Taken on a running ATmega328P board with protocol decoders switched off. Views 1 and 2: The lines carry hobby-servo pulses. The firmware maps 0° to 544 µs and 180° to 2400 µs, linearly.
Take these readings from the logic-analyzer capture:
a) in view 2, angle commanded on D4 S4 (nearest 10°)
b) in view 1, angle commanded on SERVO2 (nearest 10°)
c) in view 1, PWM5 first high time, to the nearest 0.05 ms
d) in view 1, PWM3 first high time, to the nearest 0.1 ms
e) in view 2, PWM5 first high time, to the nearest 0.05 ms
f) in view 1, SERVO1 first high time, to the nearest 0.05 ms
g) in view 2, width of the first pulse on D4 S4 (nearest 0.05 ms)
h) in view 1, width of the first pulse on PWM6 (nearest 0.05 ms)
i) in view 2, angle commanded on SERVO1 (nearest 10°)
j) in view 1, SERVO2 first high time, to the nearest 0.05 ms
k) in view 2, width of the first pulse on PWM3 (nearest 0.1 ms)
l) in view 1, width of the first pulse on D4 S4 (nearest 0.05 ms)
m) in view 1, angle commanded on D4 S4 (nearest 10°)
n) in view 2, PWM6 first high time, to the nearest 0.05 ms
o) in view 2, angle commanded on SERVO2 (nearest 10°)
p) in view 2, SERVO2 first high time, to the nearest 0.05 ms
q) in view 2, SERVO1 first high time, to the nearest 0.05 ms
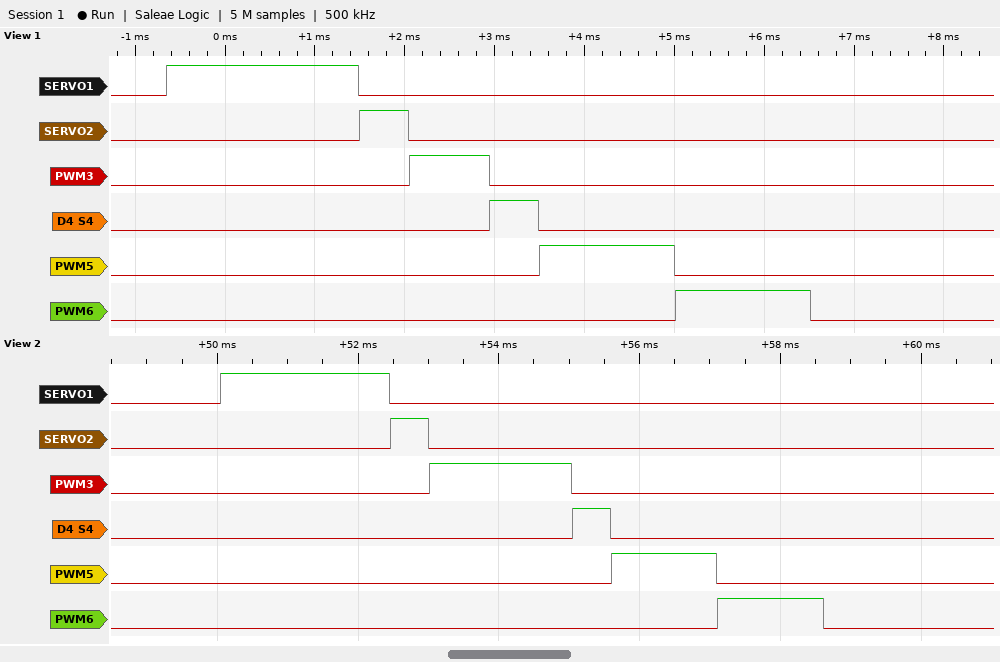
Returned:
0°
0°
1.50 ms
0.9 ms
1.50 ms
2.15 ms
0.55 ms
1.50 ms
180°
0.55 ms
2.0 ms
0.55 ms
0°
1.50 ms
0°
0.55 ms
2.40 ms
